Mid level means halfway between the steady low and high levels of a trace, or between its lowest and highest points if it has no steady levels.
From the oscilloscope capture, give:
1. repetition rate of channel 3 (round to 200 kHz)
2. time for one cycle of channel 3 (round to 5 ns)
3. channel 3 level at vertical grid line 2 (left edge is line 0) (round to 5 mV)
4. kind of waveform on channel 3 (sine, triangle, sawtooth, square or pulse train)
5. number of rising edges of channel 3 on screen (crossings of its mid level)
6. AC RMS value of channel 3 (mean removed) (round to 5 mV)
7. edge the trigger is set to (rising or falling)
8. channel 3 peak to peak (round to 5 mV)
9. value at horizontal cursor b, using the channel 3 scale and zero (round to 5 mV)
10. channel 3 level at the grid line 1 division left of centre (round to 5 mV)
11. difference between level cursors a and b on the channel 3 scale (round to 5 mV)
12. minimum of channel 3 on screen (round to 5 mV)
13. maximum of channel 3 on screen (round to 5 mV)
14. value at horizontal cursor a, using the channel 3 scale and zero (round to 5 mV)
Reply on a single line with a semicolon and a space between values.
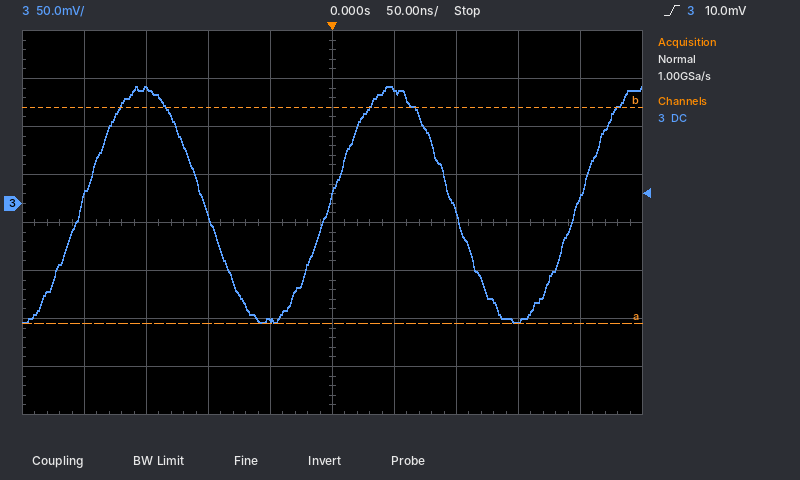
5.0 MHz; 200 ns; 120 mV; sine; 3; 85 mV; rising; 245 mV; 100 mV; -120 mV; 225 mV; -125 mV; 120 mV; -125 mV
